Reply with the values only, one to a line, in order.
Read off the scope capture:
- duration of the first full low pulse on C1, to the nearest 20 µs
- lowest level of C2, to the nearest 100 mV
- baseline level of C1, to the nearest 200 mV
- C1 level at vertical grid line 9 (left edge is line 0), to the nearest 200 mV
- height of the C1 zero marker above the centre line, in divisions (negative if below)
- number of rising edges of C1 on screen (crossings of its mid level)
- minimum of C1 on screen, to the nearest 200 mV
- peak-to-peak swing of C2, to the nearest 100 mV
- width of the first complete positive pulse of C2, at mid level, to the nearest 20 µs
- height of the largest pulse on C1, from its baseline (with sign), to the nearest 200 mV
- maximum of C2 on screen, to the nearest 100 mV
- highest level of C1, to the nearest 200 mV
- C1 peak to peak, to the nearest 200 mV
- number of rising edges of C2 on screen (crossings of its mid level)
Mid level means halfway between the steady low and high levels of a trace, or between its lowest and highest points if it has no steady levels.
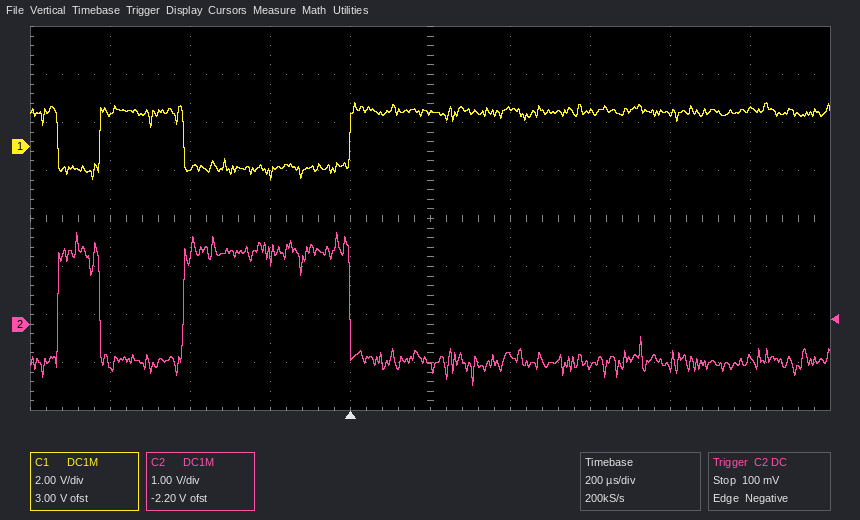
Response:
100 µs
-1.3 V
1.4 V
1.6 V
+1.5 div
2
-1.4 V
3.2 V
100 µs
-2.8 V
1.9 V
1.8 V
3.2 V
2
